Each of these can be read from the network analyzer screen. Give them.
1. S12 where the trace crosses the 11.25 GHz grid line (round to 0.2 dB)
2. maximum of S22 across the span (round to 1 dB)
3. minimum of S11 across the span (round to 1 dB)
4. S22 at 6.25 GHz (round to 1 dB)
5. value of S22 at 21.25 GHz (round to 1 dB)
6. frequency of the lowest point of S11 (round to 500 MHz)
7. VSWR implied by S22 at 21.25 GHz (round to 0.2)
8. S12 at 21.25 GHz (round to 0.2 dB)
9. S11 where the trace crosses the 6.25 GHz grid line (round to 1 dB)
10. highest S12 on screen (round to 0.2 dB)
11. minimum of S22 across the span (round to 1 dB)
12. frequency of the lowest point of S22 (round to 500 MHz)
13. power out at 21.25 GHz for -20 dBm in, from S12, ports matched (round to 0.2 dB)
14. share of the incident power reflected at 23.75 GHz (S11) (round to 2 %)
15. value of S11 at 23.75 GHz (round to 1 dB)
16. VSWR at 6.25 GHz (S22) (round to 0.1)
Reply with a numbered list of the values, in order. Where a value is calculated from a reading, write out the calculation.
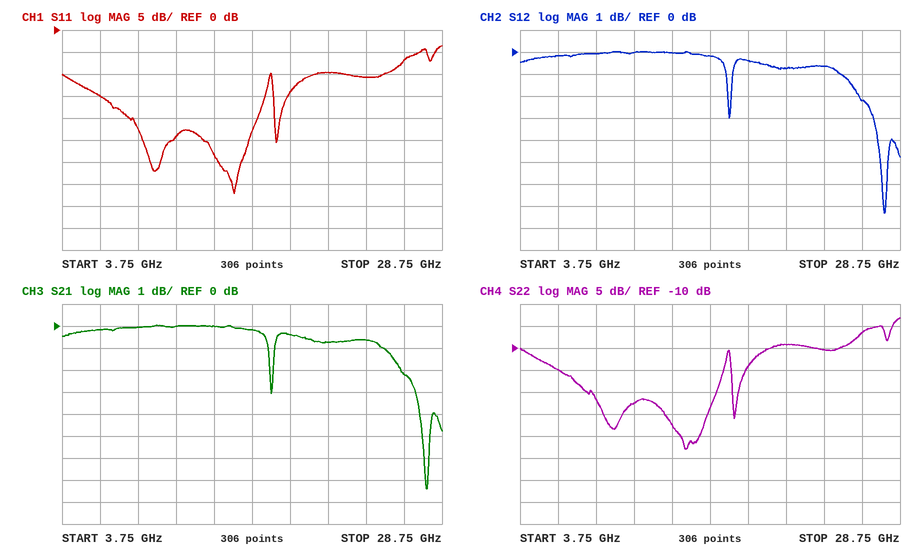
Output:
1. 0.0 dB
2. -3 dB
3. -37 dB
4. -15 dB
5. -9 dB
6. 15.0 GHz
7. |Γ| = 10^(-9/20) = 0.3548; VSWR = (1 + 0.3548)/(1 − 0.3548) ≈ 2.10, so 2.0 to the nearest 0.2
8. -0.8 dB
9. -15 dB
10. 0.0 dB
11. -33 dB
12. 14.5 GHz
13. -20 dBm + (-0.8 dB) = -20.8 dBm
14. 10^(-11/10) ≈ 8 %
15. -11 dB
16. |Γ| = 10^(-15/20) = 0.1778; VSWR = (1 + 0.1778)/(1 − 0.1778) ≈ 1.4
